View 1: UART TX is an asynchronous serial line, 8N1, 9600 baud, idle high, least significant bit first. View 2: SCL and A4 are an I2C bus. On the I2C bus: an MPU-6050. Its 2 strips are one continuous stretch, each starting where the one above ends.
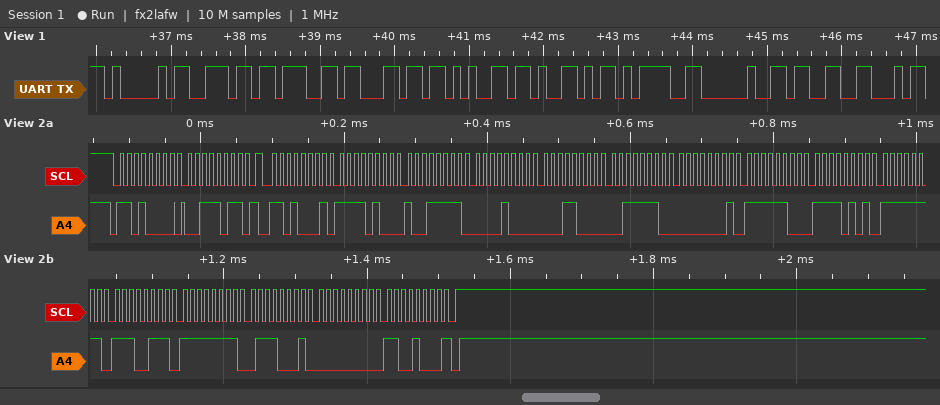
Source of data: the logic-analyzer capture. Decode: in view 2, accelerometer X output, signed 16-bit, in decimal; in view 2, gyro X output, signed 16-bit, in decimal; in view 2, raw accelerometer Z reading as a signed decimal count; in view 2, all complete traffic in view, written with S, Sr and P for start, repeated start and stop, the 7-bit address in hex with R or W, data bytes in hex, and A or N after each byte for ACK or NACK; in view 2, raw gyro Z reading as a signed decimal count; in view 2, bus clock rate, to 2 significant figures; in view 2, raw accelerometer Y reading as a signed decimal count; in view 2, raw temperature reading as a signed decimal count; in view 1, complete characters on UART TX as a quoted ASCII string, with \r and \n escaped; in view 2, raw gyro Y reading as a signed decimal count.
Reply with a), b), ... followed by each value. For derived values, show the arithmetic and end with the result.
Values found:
a) 0xF49F = -2913
b) 0xFFE7 = -25
c) 0x3E01 = 15873
d) S 68W A 3B A Sr 68R A F4 A 9F A 08 A 18 A 3E A 01 A FC A F5 A FF A E7 A FF A 71 A 00 A C8 N P
e) 0x00C8 = 200
f) 100 kHz
g) 0x0818 = 2072
h) 0xFCF5 = -779
i) "AngleY= 3"
j) 0xFF71 = -143
